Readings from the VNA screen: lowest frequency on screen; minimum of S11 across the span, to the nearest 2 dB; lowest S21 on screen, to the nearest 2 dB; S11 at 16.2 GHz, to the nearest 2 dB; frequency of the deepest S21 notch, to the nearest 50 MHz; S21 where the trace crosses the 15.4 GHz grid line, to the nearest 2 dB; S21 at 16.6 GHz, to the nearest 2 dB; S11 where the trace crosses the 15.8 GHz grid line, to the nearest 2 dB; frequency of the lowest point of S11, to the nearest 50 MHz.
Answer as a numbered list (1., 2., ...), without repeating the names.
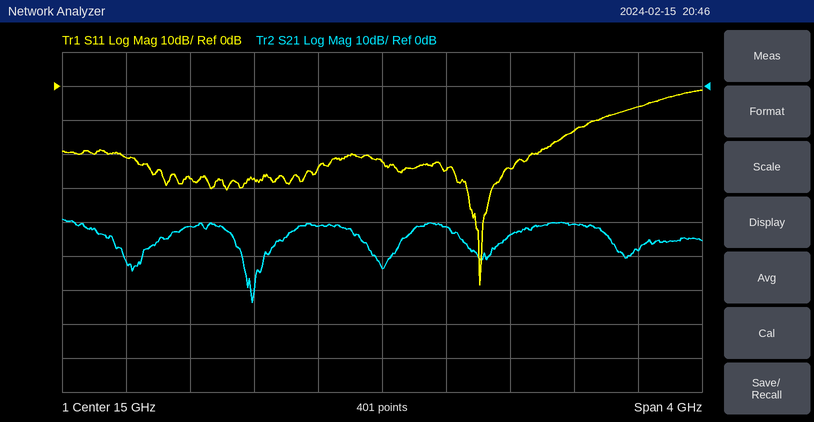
1. 13 GHz
2. -58 dB
3. -64 dB
4. -14 dB
5. 14.20 GHz
6. -42 dB
7. -48 dB
8. -24 dB
9. 15.60 GHz
